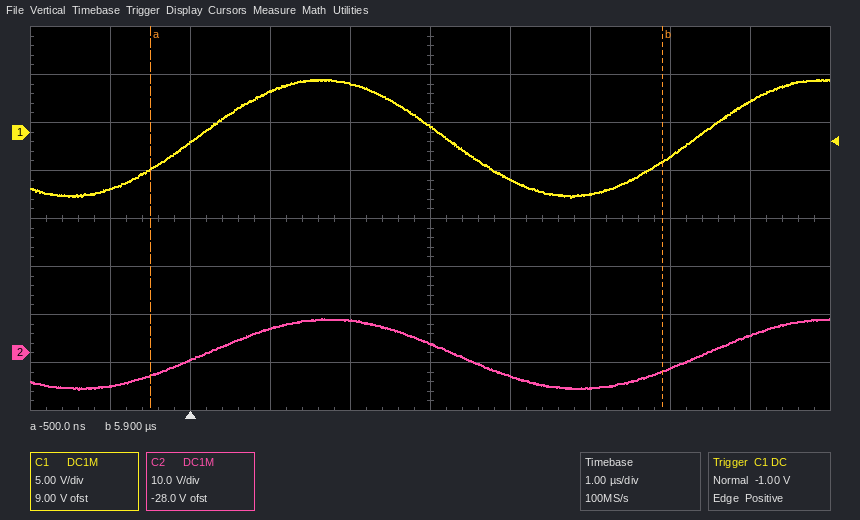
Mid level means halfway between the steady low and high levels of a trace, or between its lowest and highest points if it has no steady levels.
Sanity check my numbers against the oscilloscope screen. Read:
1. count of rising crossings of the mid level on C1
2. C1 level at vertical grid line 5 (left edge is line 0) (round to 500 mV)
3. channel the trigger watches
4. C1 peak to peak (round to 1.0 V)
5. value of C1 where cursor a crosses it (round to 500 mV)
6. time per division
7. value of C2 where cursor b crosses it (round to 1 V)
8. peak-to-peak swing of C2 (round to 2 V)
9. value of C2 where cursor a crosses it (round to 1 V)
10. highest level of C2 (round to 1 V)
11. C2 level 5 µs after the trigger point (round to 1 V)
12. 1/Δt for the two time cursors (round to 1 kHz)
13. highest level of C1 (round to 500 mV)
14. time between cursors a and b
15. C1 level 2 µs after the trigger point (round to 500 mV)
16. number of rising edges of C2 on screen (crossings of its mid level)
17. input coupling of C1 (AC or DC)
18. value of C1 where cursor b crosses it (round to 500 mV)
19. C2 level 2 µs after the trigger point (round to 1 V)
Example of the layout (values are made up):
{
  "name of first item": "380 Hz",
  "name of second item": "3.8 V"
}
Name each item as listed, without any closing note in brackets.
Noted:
{
  "count of rising crossings of the mid level on C1": "2",
  "C1 level at vertical grid line 5 (left edge is line 0)": "500 mV",
  "channel the trigger watches": "C1",
  "C1 peak to peak": "12.0 V",
  "value of C1 where cursor a crosses it": "-4.0 V",
  "time per division": "1 µs",
  "value of C2 where cursor b crosses it": "-4 V",
  "peak-to-peak swing of C2": "14 V",
  "value of C2 where cursor a crosses it": "-5 V",
  "highest level of C2": "7 V",
  "C2 level 5 µs after the trigger point": "-7 V",
  "1/Δt for the two time cursors": "156 kHz",
  "highest level of C1": "5.5 V",
  "time between cursors a and b": "6.4 µs",
  "C1 level 2 µs after the trigger point": "5.0 V",
  "number of rising edges of C2 on screen": "2",
  "input coupling of C1": "DC",
  "value of C1 where cursor b crosses it": "-3.0 V",
  "C2 level 2 µs after the trigger point": "7 V"
}
